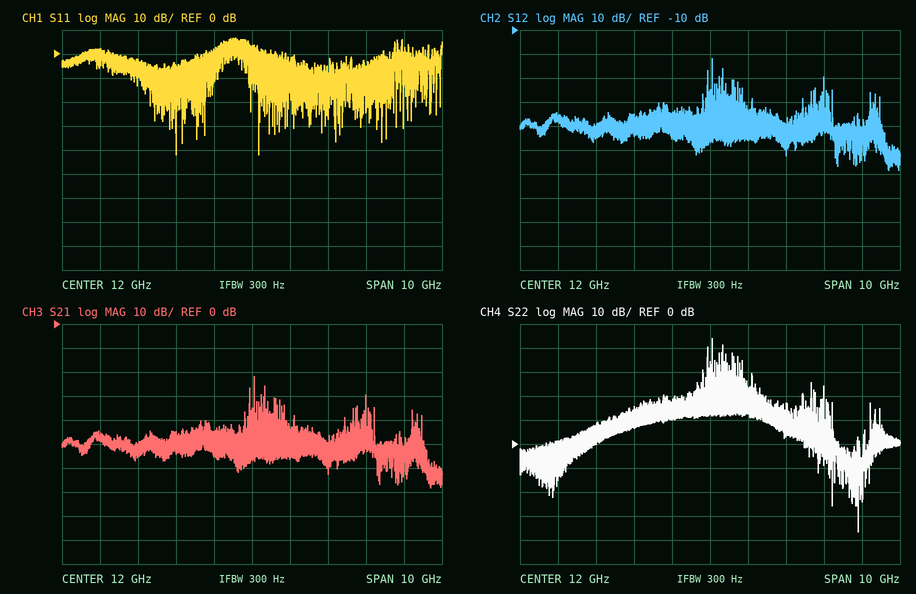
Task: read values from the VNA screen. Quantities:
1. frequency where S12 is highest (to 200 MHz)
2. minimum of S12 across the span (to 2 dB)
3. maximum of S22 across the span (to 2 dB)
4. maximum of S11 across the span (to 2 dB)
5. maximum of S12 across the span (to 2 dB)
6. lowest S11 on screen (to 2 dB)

12.0 GHz
-68 dB
44 dB
6 dB
-22 dB
-42 dB
